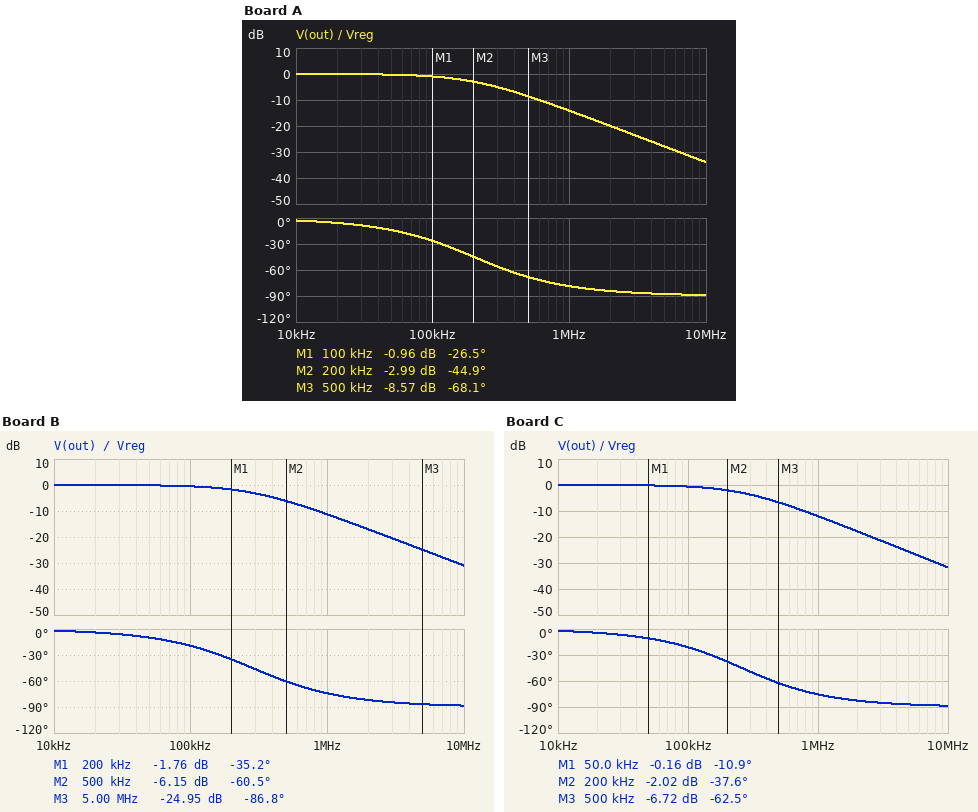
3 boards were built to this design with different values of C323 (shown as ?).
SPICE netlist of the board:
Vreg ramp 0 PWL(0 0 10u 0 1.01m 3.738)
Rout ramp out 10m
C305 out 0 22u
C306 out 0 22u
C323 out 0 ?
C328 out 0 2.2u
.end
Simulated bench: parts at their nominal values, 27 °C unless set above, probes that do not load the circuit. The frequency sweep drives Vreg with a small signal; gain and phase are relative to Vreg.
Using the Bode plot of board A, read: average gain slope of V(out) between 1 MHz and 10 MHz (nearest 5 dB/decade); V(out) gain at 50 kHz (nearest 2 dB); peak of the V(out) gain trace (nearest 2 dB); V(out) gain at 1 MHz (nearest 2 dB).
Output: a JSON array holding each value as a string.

["-20 dB/decade", "0 dB", "0 dB", "-14 dB"]
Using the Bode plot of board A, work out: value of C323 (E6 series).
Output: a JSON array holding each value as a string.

["33 µF"]
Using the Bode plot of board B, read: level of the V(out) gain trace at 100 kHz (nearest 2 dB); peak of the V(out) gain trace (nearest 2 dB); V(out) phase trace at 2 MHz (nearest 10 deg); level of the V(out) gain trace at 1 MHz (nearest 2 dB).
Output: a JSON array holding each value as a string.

["0 dB", "0 dB", "-80 deg", "-12 dB"]
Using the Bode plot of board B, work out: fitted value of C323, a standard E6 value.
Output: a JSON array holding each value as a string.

["10 µF"]
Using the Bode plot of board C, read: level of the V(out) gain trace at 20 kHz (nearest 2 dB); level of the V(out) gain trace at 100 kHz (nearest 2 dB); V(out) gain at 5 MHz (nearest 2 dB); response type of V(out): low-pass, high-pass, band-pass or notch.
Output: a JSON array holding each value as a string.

["0 dB", "0 dB", "-26 dB", "low-pass"]
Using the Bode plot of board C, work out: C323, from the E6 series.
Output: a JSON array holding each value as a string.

["15 µF"]
